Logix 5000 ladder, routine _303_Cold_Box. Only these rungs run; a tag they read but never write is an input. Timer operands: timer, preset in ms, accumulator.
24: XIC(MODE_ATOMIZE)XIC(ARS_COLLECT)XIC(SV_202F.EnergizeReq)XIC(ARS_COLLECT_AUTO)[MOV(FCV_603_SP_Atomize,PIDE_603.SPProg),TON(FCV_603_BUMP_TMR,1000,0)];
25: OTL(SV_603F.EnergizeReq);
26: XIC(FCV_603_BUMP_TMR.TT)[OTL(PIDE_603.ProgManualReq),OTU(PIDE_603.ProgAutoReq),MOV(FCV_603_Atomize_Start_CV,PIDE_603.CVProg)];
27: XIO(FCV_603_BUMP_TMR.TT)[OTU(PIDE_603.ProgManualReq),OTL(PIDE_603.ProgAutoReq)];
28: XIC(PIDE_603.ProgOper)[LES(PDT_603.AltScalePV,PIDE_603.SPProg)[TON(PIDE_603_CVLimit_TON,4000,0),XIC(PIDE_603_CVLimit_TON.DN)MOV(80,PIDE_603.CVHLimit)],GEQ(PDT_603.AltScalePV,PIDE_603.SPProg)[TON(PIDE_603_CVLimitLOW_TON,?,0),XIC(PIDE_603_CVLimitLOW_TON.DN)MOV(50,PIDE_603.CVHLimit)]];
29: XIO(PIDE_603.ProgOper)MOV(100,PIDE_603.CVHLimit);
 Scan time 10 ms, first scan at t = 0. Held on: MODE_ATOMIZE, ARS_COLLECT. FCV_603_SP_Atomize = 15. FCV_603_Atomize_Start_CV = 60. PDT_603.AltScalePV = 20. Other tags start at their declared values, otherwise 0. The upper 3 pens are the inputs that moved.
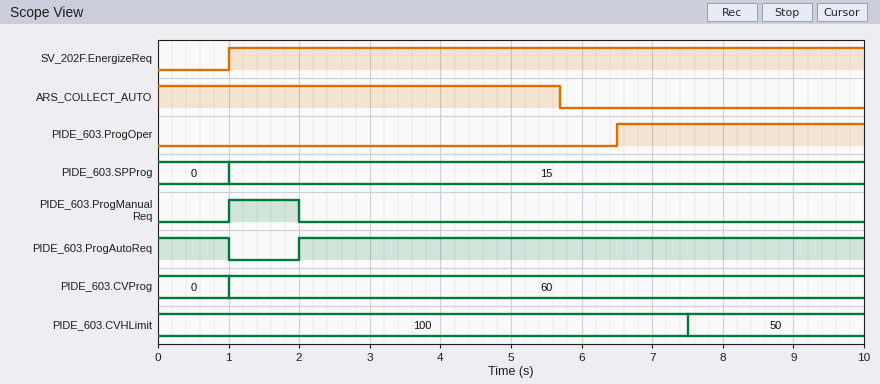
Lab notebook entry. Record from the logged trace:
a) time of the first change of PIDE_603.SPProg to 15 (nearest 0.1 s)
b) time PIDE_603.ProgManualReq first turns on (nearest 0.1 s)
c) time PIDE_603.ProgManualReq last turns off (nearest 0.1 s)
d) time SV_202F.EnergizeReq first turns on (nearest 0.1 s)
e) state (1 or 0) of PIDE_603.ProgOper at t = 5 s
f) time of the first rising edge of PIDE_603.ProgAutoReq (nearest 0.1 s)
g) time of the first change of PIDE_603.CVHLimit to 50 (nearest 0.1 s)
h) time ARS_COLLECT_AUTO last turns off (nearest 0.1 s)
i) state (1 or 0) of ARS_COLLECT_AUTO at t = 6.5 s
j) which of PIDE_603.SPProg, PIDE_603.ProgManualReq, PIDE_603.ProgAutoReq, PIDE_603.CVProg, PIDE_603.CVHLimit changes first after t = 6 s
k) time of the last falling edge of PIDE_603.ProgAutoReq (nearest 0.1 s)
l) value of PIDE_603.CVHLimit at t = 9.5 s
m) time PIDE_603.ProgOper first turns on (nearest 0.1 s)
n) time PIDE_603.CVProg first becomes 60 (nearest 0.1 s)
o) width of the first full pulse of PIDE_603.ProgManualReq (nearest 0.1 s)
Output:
1.0 s
1.0 s
2.0 s
1.0 s
0
2.0 s
7.5 s
5.7 s
0
PIDE_603.CVHLimit
1.0 s
50
6.5 s
1.0 s
1.0 s
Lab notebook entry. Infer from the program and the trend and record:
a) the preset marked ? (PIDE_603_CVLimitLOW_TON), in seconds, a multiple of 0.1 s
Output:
1.0 s
